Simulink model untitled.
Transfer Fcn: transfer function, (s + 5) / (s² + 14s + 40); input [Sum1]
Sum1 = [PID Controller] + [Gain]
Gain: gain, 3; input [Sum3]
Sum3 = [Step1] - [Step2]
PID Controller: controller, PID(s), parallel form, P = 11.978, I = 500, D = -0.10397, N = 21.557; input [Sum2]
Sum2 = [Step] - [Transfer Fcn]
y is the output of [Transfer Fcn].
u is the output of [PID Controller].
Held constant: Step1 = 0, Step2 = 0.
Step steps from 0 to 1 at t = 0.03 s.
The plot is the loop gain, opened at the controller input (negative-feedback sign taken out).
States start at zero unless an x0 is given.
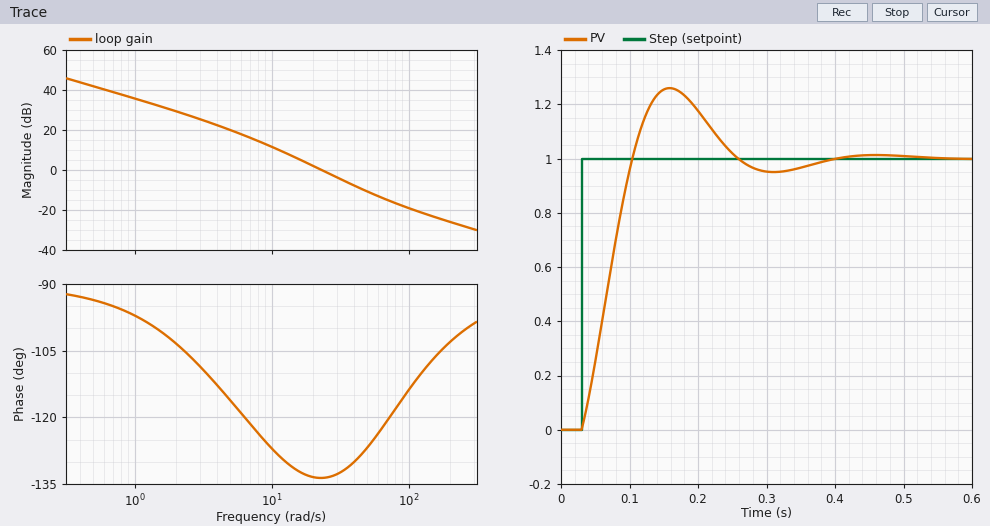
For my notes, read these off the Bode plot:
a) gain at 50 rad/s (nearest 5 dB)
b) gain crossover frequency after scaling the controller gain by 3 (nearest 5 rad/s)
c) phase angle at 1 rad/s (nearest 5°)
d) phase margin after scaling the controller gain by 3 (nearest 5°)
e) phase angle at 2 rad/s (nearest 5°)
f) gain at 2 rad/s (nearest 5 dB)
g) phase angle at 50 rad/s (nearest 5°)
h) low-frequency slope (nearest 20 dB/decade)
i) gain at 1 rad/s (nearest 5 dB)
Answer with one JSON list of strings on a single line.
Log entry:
["-10 dB", "45 rad/s", "-95°", "50°", "-105°", "30 dB", "-125°", "-20 dB/decade", "35 dB"]
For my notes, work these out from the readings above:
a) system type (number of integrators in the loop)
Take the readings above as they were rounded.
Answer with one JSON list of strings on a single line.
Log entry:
["1"]
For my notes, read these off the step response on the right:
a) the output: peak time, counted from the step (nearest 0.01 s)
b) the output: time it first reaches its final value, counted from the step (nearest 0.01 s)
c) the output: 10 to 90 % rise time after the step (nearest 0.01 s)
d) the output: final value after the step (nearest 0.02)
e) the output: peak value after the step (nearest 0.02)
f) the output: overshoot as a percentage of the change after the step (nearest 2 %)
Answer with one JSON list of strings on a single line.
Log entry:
["0.13 s", "0.07 s", "0.06 s", "1.00", "1.26", "26 %"]
